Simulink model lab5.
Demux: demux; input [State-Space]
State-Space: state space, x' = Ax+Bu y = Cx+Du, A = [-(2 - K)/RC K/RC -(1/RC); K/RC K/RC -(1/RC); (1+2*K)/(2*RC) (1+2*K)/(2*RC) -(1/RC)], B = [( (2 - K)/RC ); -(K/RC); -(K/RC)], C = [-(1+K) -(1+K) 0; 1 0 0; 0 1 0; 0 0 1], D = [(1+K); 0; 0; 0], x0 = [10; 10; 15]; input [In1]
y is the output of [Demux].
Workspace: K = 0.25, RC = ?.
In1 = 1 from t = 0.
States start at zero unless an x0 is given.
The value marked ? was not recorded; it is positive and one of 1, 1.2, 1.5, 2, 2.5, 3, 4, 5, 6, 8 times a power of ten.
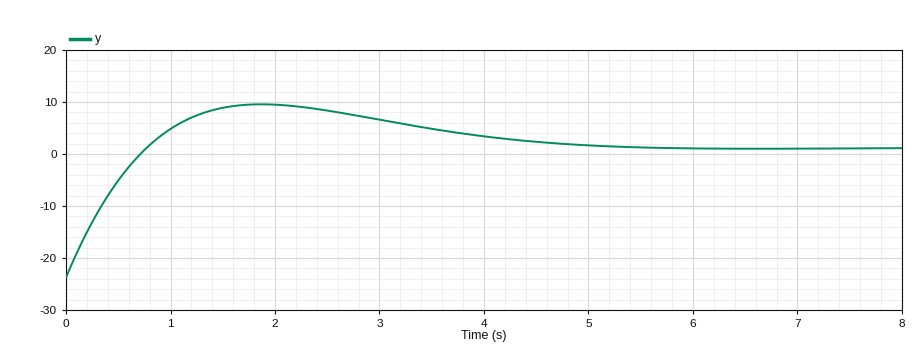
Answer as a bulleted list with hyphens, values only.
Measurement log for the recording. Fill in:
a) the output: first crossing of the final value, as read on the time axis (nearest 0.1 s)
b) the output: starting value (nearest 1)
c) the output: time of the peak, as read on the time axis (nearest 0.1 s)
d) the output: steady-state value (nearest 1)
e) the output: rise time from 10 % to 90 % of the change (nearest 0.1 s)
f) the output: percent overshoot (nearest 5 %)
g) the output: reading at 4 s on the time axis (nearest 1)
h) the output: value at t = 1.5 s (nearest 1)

- 0.8 s
- -24
- 1.9 s
- 1
- 0.6 s
- 35 %
- 3
- 9
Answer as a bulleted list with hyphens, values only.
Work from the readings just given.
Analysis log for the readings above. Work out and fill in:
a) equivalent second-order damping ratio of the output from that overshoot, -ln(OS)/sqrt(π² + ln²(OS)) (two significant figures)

- 0.32
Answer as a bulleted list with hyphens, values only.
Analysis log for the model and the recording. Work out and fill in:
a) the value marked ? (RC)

- 1
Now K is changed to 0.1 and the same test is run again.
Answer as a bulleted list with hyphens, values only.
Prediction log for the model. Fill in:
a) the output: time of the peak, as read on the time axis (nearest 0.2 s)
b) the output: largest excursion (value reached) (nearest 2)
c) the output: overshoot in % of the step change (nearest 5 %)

- 1.8 s
- 8
- 30 %
